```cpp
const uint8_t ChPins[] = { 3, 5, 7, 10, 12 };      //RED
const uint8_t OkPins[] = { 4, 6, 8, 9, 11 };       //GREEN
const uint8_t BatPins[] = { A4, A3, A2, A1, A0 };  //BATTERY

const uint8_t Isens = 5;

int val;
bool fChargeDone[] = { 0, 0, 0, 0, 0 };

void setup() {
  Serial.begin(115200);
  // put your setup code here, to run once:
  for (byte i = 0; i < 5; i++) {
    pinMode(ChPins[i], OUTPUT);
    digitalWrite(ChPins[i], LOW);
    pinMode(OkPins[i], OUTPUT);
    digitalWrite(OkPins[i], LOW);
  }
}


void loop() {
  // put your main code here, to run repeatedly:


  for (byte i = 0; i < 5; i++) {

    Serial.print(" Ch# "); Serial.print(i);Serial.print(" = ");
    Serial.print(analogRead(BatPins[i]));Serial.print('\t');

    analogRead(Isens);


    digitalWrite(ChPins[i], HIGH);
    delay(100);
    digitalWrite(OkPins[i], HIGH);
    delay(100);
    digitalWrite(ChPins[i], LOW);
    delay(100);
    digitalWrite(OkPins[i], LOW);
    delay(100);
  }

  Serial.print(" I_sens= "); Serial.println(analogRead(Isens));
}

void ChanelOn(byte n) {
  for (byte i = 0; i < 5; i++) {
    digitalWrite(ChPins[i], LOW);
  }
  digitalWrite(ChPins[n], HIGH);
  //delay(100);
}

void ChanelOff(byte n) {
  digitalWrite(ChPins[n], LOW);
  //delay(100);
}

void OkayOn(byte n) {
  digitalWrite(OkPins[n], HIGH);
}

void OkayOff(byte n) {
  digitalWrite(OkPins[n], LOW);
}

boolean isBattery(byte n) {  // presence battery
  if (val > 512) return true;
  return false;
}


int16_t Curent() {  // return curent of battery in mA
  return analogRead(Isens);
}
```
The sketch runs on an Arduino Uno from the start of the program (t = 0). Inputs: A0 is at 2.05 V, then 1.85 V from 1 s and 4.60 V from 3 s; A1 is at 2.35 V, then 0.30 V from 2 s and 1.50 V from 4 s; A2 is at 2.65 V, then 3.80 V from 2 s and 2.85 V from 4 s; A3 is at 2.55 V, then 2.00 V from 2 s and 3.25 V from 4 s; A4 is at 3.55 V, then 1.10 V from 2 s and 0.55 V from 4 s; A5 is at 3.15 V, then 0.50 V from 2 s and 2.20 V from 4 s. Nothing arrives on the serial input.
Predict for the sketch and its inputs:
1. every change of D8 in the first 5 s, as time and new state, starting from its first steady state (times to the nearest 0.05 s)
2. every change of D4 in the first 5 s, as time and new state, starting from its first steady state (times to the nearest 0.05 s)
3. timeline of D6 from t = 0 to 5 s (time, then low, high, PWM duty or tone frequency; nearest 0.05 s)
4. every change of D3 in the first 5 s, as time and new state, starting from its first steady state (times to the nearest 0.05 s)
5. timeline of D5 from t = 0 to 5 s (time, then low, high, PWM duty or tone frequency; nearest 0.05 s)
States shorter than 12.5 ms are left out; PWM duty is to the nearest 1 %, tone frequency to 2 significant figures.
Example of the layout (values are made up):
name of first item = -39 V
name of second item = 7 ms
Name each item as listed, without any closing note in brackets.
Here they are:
every change of D8 in the first 5 s, as time and new state, starting from its first steady state = 0 s low; 0.9 s high; 1.1 s low; 2.9 s high; 3.1 s low; 4.9 s high
every change of D4 in the first 5 s, as time and new state, starting from its first steady state = 0 s low; 0.1 s high; 0.3 s low; 2.1 s high; 2.3 s low; 4.1 s high; 4.3 s low
timeline of D6 from t = 0 to 5 s = 0 s low; 0.5 s high; 0.7 s low; 2.5 s high; 2.7 s low; 4.5 s high; 4.7 s low
every change of D3 in the first 5 s, as time and new state, starting from its first steady state = 0 s high; 0.2 s low; 2 s high; 2.2 s low; 4 s high; 4.2 s low
timeline of D5 from t = 0 to 5 s = 0 s low; 0.4 s high; 0.6 s low; 2.4 s high; 2.6 s low; 4.4 s high; 4.6 s low
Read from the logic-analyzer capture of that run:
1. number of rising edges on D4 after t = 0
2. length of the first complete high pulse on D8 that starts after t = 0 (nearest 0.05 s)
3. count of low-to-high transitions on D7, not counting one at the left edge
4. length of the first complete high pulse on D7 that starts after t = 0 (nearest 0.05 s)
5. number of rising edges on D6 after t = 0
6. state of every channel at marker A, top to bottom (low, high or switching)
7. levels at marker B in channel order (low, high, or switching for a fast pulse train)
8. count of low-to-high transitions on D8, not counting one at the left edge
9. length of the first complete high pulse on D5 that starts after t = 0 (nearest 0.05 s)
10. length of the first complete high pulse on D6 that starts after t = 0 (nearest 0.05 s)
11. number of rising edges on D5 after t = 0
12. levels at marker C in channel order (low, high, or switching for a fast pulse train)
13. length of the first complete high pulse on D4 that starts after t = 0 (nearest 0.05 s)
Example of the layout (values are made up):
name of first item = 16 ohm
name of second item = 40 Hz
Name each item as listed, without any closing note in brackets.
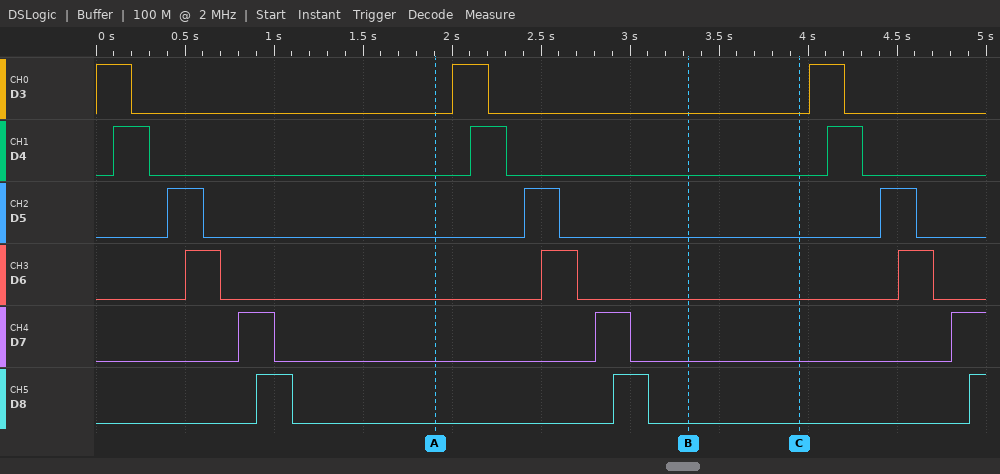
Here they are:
number of rising edges on D4 after t = 0 = 3
length of the first complete high pulse on D8 that starts after t = 0 = 0.20 s
count of low-to-high transitions on D7, not counting one at the left edge = 3
length of the first complete high pulse on D7 that starts after t = 0 = 0.20 s
number of rising edges on D6 after t = 0 = 3
state of every channel at marker A, top to bottom = D3 low, D4 low, D5 low, D6 low, D7 low, D8 low
levels at marker B in channel order = D3 low, D4 low, D5 low, D6 low, D7 low, D8 low
count of low-to-high transitions on D8, not counting one at the left edge = 3
length of the first complete high pulse on D5 that starts after t = 0 = 0.20 s
length of the first complete high pulse on D6 that starts after t = 0 = 0.20 s
number of rising edges on D5 after t = 0 = 3
levels at marker C in channel order = D3 low, D4 low, D5 low, D6 low, D7 low, D8 low
length of the first complete high pulse on D4 that starts after t = 0 = 0.20 s
